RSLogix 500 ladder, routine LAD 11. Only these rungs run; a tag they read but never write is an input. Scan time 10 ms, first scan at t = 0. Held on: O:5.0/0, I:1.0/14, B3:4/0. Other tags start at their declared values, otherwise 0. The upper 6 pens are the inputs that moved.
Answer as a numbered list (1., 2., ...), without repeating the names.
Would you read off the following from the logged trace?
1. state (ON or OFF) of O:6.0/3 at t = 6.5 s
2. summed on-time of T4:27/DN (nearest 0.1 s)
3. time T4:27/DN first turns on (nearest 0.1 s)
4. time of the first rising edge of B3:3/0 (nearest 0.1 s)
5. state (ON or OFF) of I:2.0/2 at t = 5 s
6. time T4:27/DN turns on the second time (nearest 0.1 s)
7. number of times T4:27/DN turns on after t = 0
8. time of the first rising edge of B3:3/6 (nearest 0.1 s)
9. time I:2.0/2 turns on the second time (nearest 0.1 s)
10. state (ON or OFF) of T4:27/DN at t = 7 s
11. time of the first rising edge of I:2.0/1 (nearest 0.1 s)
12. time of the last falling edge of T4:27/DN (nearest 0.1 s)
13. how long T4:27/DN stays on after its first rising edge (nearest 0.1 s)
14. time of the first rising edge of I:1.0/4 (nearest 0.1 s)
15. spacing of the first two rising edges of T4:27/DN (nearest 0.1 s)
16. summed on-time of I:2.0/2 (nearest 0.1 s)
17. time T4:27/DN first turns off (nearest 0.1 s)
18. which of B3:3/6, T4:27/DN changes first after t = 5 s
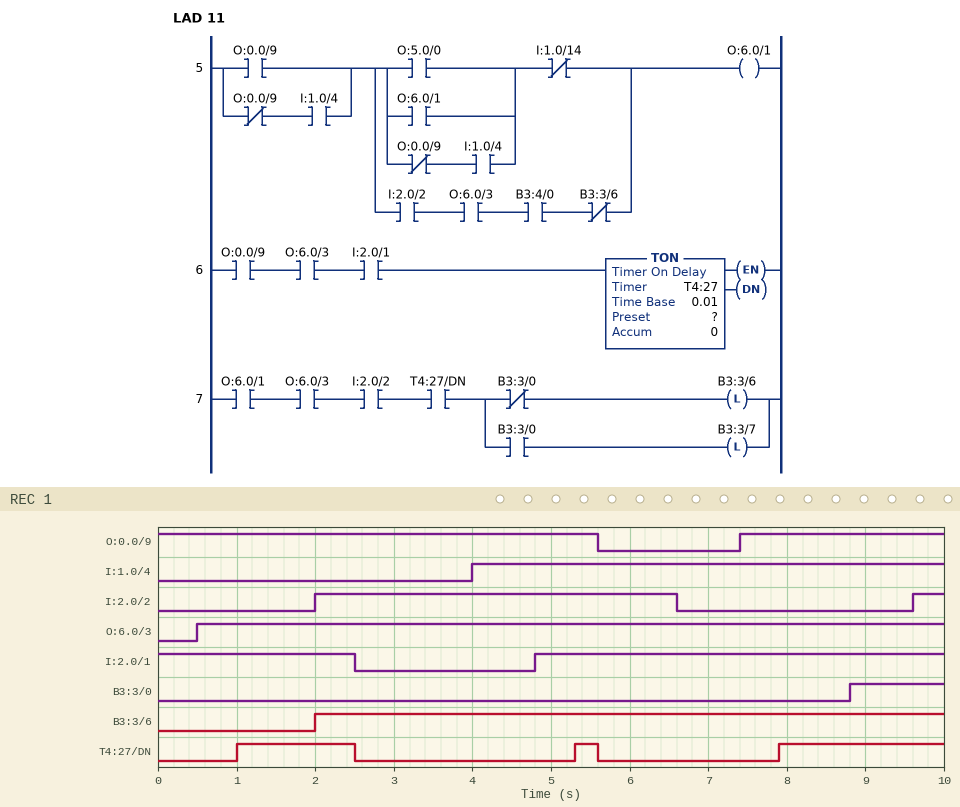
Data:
1. ON
2. 3.9 s
3. 1.0 s
4. 8.8 s
5. ON
6. 5.3 s
7. 3
8. 2.0 s
9. 9.6 s
10. OFF
11. 4.8 s
12. 5.6 s
13. 1.5 s
14. 4.0 s
15. 4.3 s
16. 5.0 s
17. 2.5 s
18. T4:27/DN
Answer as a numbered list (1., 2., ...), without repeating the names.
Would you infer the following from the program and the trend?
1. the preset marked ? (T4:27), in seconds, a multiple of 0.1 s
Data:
1. 0.5 s
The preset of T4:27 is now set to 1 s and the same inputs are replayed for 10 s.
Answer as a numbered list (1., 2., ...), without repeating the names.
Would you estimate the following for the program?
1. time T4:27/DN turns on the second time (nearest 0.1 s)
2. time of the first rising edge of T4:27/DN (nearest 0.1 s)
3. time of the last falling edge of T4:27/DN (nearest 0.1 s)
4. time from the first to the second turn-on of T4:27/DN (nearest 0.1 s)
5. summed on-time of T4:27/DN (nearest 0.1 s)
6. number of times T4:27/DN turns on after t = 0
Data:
1. 8.4 s
2. 1.5 s
3. 2.5 s
4. 6.9 s
5. 2.6 s
6. 2
